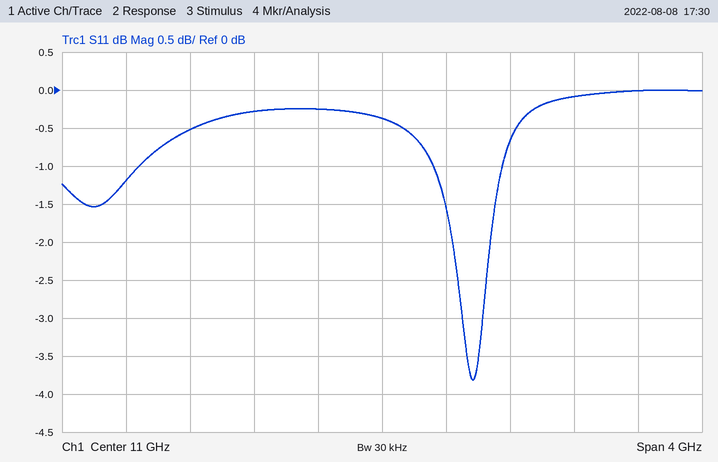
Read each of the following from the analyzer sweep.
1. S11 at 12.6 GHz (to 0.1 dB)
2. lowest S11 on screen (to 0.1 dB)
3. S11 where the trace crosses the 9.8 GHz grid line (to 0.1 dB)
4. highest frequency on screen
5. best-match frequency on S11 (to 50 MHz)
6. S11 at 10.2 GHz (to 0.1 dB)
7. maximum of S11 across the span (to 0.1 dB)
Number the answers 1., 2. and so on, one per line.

1. 0.0 dB
2. -3.8 dB
3. -0.5 dB
4. 13 GHz
5. 11.55 GHz
6. -0.3 dB
7. 0.0 dB
